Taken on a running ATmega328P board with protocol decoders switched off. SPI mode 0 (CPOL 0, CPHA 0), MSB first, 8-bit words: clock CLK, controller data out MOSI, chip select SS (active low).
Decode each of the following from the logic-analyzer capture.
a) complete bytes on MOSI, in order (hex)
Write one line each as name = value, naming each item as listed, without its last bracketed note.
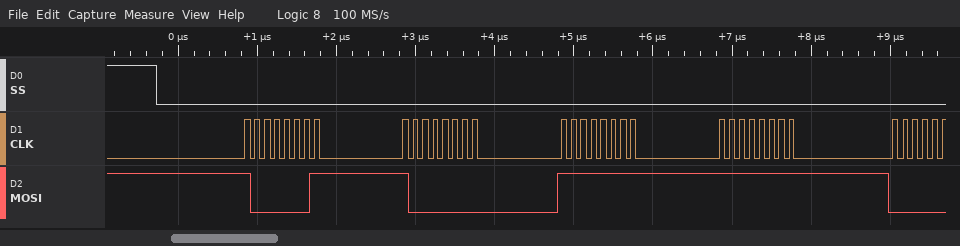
complete bytes on MOSI, in order = 81 80 FF FF
